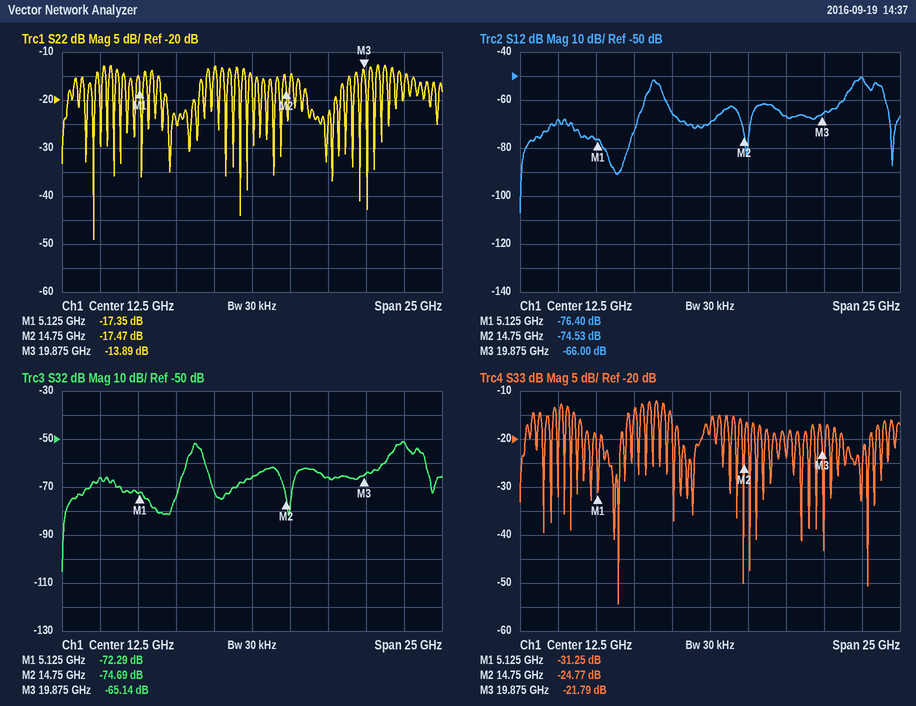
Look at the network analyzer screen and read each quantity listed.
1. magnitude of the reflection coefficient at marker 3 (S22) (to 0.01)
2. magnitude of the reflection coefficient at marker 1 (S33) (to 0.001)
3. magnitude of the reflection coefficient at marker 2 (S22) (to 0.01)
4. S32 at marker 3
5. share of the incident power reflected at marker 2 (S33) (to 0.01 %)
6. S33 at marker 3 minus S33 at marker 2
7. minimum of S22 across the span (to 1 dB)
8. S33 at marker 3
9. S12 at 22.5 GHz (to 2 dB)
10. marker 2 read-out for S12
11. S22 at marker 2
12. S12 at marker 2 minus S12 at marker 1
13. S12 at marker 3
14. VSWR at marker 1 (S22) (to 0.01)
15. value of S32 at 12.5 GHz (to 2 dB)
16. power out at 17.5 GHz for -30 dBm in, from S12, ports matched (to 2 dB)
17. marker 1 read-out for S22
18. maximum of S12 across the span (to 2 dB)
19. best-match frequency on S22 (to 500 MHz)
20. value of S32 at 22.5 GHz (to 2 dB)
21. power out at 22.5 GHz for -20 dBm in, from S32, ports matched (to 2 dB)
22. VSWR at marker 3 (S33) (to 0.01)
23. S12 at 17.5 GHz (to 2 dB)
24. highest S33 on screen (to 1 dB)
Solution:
0.20
0.027
0.13
-65.14 dB
0.33 %
2.98 dB
-49 dB
-21.79 dB
-50 dB
-74.53 dB
-17.47 dB
1.87 dB
-66.00 dB
1.31
-66 dB
-96 dBm
-17.35 dB
-50 dB
2.0 GHz
-52 dB
-72 dBm
1.18
-66 dB
-12 dB
